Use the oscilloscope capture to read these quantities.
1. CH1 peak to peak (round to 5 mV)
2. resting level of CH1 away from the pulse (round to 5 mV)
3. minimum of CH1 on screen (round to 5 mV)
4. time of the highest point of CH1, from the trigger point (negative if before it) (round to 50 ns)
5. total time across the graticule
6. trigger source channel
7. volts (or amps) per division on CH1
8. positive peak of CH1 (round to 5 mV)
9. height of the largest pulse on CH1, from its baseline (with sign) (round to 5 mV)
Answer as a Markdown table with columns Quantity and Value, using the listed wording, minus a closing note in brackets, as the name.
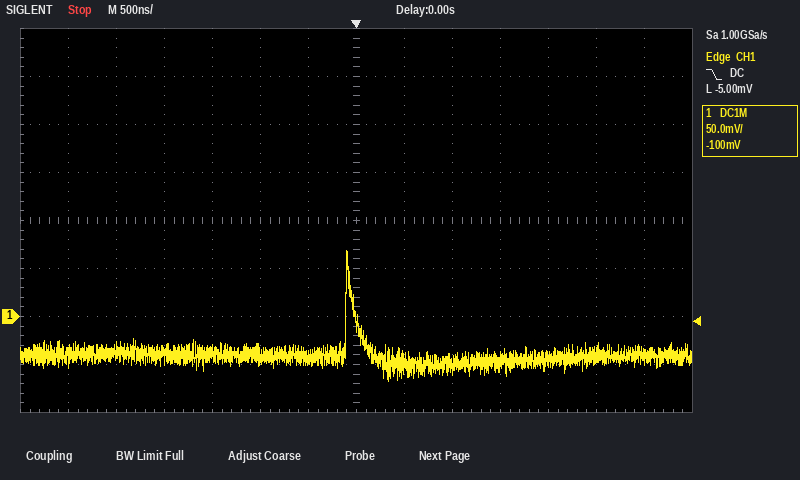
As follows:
| Quantity | Value |
|---|---|
| CH1 peak to peak | 135 mV |
| resting level of CH1 away from the pulse | -40 mV |
| minimum of CH1 on screen | -65 mV |
| time of the highest point of CH1, from the trigger point (negative if before it) | -100 ns |
| total time across the graticule | 7 µs |
| trigger source channel | CH1 |
| volts (or amps) per division on CH1 | 50 mV |
| positive peak of CH1 | 70 mV |
| height of the largest pulse on CH1, from its baseline (with sign) | +110 mV |
